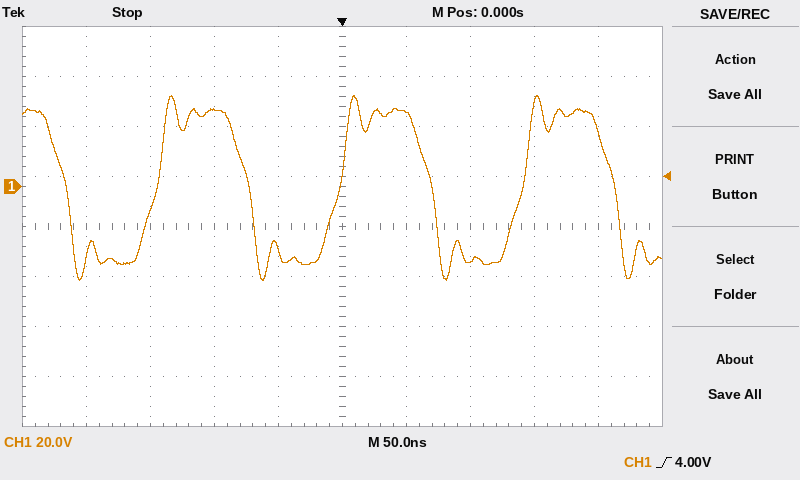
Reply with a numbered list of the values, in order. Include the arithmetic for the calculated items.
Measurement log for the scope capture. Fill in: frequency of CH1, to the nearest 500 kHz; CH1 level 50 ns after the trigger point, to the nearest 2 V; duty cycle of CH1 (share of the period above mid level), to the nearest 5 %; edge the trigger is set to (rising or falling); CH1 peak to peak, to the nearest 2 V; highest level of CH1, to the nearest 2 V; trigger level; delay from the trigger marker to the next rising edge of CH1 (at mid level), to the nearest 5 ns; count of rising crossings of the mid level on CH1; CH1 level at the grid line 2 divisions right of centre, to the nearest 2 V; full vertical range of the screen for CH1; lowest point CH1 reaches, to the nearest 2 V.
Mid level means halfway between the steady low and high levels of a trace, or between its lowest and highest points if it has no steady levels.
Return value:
1. 7.0 MHz
2. 30 V
3. 50 %
4. rising
5. 36 V − (-38 V) = 74 V
6. 36 V
7. 4.00 V
8. 140 ns
9. 3
10. -30 V
11. 160 V
12. -38 V
